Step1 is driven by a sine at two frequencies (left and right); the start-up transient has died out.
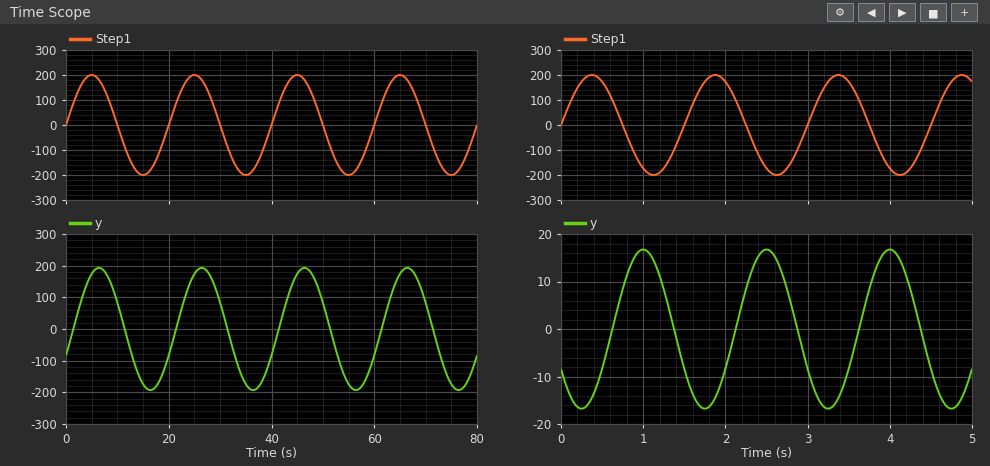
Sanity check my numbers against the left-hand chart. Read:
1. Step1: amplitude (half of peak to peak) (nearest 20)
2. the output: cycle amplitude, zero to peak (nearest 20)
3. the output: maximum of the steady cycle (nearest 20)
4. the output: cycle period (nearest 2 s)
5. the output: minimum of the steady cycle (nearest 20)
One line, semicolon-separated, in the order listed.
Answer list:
200; 200; 200; 20 s; -200
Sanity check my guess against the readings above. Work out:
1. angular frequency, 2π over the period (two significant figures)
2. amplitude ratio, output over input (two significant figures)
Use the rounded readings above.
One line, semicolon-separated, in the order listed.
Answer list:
0.31 rad/s; 1.0
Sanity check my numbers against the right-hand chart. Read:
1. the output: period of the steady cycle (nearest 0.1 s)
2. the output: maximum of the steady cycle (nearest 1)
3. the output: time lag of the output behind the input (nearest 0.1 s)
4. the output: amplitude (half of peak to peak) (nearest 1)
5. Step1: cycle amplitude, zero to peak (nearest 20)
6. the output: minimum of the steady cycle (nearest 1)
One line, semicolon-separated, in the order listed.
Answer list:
1.5 s; 17; 0.6 s; 17; 200; -17
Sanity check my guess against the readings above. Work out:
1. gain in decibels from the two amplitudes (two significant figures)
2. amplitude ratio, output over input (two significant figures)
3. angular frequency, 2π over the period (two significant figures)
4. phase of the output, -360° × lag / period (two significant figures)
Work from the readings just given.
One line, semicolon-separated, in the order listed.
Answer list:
-21 dB; 0.085; 4.2 rad/s; -140°
